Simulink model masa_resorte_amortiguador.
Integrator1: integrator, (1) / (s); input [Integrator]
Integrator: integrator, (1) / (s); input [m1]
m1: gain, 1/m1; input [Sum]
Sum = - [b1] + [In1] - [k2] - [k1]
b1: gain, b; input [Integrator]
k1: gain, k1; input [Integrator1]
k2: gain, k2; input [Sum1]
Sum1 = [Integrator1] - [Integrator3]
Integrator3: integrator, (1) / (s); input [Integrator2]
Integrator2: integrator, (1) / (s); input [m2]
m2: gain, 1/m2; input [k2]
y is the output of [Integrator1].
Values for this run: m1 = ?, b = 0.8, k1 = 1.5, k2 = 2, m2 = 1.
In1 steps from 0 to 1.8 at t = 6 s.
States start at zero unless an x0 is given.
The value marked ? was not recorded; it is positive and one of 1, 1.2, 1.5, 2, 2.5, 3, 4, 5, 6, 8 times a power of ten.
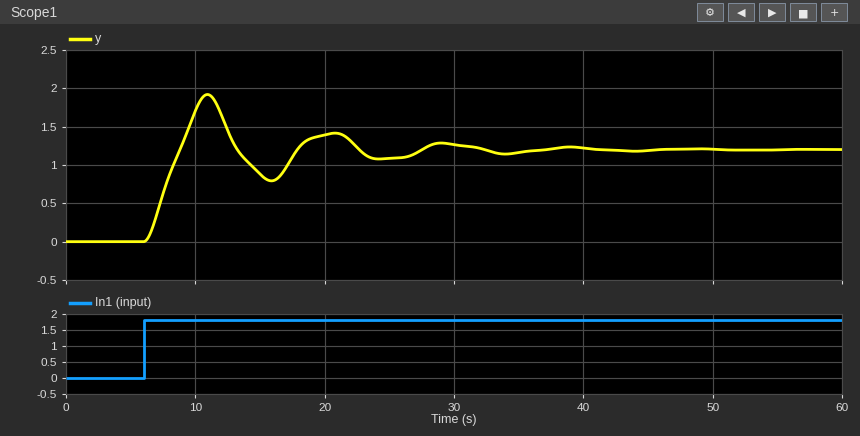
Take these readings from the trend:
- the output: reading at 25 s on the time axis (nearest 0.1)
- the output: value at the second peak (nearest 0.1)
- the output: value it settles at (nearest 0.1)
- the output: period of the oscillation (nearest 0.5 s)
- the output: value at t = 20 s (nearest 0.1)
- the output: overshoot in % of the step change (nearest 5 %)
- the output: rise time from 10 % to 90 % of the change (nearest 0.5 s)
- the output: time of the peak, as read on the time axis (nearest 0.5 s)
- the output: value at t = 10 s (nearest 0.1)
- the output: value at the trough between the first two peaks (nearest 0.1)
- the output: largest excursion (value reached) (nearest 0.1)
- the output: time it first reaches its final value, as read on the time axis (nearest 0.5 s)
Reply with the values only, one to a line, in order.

1.1
1.4
1.2
10.0 s
1.4
60 %
2.0 s
11.0 s
1.7
0.8
1.9
9.0 s
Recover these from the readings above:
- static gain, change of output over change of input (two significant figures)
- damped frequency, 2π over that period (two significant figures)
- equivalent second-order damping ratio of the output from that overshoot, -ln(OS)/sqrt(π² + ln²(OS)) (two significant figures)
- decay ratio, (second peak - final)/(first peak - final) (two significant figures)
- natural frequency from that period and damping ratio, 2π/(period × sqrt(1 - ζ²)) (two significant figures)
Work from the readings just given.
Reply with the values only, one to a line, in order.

0.67
0.63 rad/s
0.16
0.29
0.64 rad/s
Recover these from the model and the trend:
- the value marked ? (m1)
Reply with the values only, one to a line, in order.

2
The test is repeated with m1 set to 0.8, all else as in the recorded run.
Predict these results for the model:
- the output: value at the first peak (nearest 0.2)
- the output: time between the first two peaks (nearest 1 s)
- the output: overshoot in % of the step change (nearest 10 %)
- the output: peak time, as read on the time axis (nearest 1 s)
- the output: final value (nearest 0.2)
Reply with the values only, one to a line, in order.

1.8
8 s
50 %
10 s
1.2
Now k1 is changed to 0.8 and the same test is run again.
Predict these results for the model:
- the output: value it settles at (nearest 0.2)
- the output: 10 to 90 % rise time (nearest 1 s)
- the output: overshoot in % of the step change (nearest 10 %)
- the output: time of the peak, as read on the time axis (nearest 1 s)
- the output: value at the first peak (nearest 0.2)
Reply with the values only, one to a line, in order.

2.2
3 s
40 %
12 s
3.2
